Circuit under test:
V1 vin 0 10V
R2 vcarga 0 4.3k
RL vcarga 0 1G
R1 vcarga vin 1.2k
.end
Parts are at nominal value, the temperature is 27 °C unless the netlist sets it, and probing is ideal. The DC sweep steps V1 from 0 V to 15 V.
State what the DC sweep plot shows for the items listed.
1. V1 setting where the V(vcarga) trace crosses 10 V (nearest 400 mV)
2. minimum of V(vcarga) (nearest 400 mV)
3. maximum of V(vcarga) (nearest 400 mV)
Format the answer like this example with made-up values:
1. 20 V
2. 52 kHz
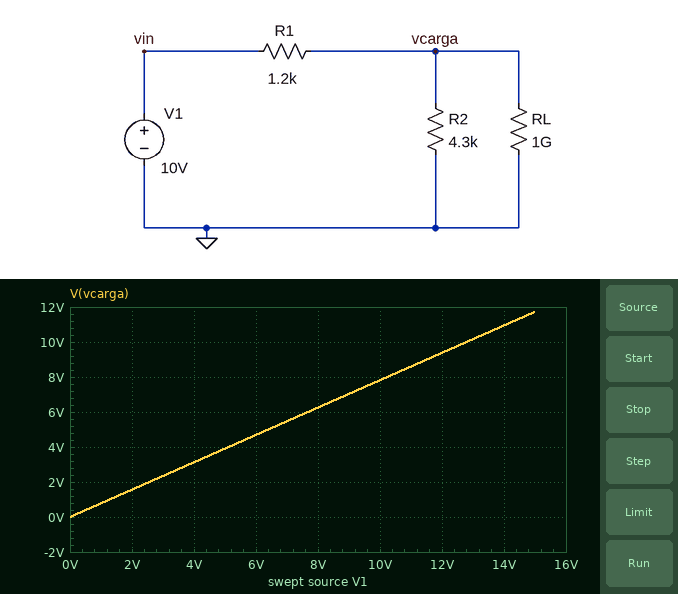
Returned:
1. 12.8 V
2. 0 V
3. 11.6 V
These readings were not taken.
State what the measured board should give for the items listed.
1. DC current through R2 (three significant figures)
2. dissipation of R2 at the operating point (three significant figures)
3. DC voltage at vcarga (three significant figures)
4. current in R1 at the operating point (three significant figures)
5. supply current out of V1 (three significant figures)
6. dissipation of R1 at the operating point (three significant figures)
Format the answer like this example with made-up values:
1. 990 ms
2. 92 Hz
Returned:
1. 1.82 mA
2. 14.2 mW
3. 7.82 V
4. 1.82 mA
5. 1.82 mA
6. 3.97 mW
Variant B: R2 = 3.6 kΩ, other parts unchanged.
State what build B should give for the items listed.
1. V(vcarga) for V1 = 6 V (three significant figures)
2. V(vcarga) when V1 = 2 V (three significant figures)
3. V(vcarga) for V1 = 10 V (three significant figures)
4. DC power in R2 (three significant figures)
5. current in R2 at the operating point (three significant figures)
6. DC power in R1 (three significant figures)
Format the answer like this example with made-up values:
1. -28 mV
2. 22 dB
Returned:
1. 4.50 V
2. 1.50 V
3. 7.50 V
4. 15.6 mW
5. 2.08 mA
6. 5.21 mW
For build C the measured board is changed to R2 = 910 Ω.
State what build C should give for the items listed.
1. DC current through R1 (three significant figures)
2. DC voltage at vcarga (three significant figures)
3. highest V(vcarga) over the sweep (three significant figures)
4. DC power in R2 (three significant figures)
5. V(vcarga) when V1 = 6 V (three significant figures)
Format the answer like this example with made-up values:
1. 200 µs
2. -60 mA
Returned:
1. 4.74 mA
2. 4.31 V
3. 6.47 V
4. 20.4 mW
5. 2.59 V
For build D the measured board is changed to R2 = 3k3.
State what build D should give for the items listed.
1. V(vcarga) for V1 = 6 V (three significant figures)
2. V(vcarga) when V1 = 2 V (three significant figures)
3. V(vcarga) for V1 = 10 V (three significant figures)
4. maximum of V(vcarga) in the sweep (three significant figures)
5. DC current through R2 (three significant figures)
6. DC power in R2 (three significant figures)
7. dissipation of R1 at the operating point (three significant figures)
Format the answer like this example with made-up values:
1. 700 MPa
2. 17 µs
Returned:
1. 4.40 V
2. 1.47 V
3. 7.33 V
4. 11.0 V
5. 2.22 mA
6. 16.3 mW
7. 5.93 mW
